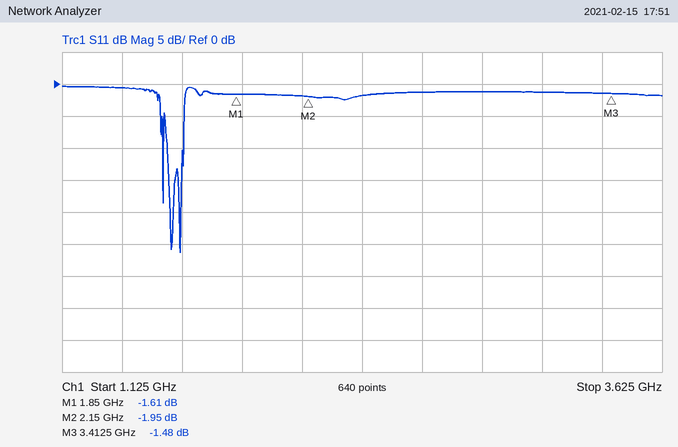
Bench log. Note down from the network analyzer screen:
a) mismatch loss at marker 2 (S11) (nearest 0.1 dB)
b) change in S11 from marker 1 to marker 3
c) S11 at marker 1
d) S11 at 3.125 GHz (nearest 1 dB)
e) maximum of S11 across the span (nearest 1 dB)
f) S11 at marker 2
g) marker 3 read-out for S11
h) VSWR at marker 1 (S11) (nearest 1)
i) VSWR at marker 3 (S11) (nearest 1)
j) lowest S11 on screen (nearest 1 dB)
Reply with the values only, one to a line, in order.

4.4 dB
0.13 dB
-1.61 dB
-1 dB
0 dB
-1.95 dB
-1.48 dB
11
12
-26 dB
